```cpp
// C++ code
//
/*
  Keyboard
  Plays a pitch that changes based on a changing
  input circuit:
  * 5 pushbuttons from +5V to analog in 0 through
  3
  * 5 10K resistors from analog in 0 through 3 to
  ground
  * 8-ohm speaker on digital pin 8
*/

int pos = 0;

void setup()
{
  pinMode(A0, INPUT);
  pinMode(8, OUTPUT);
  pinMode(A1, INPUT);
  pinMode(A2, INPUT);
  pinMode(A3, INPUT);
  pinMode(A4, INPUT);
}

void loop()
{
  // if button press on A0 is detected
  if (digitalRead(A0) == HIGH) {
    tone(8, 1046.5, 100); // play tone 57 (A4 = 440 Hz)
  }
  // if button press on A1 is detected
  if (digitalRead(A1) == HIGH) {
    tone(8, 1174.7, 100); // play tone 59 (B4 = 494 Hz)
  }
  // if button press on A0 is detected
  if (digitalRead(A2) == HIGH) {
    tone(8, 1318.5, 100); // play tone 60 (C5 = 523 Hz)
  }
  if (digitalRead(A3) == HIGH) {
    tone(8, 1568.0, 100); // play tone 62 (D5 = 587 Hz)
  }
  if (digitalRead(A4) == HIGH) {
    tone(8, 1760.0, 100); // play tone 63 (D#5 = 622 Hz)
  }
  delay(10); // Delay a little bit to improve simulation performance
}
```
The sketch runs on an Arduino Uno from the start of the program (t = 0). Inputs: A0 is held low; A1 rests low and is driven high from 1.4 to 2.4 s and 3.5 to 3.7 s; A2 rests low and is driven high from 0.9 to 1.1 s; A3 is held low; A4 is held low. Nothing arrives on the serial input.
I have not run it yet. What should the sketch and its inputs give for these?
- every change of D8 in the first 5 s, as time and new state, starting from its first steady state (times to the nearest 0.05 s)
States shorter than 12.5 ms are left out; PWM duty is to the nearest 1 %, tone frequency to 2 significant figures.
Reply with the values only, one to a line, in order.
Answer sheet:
0 s low; 0.9 s tone 1300 Hz; 1.2 s low; 1.4 s tone 1200 Hz; 2.5 s low; 3.5 s tone 1200 Hz; 3.8 s low
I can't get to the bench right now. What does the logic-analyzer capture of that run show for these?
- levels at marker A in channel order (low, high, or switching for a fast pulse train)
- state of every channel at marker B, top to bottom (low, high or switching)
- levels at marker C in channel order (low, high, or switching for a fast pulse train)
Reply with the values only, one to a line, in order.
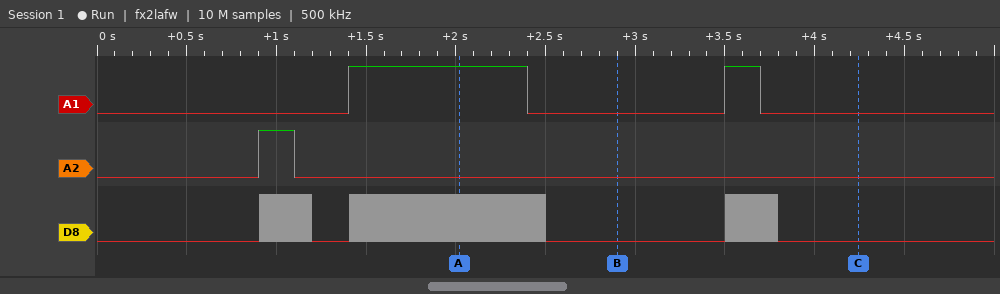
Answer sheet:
A1 high, A2 low, D8 switching
A1 low, A2 low, D8 low
A1 low, A2 low, D8 low
